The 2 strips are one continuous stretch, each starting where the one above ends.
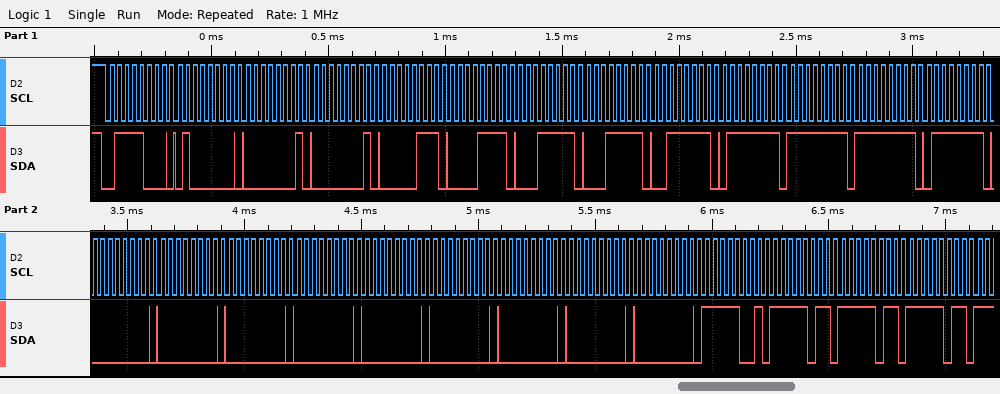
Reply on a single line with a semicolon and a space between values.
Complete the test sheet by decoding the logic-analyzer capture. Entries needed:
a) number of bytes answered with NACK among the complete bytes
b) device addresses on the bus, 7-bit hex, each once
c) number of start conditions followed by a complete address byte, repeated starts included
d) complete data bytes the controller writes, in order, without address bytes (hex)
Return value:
0; 0x3C; 1; 40 01 01 07 0F 1F 1F 3F 7F FF FF 7F 00 00 00 00 00 00 00 00 00 F9 FB FB FB
